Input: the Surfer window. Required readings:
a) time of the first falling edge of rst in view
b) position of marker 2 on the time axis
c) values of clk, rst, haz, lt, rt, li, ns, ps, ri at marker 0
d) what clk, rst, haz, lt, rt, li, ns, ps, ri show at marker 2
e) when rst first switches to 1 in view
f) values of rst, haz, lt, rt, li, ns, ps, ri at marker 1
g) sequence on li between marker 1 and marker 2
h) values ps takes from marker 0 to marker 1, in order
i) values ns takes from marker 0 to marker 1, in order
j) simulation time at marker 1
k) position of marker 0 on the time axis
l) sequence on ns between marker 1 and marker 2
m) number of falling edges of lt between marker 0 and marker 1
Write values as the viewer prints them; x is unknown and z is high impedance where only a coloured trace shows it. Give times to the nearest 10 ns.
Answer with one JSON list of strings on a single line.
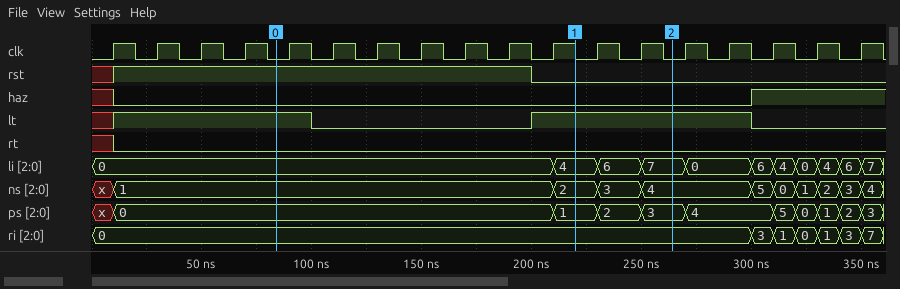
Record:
["200 ns", "260 ns", "clk=0, rst=1, haz=0, lt=1, rt=0, li=0, ns=1, ps=0, ri=0", "clk=0, rst=0, haz=0, lt=1, rt=0, li=7, ns=4, ps=3, ri=0", "10 ns", "rst=0, haz=0, lt=1, rt=0, li=4, ns=2, ps=1, ri=0", "4, 6, 7", "0, 1", "1, 2", "220 ns", "80 ns", "2, 3, 4", "1"]
